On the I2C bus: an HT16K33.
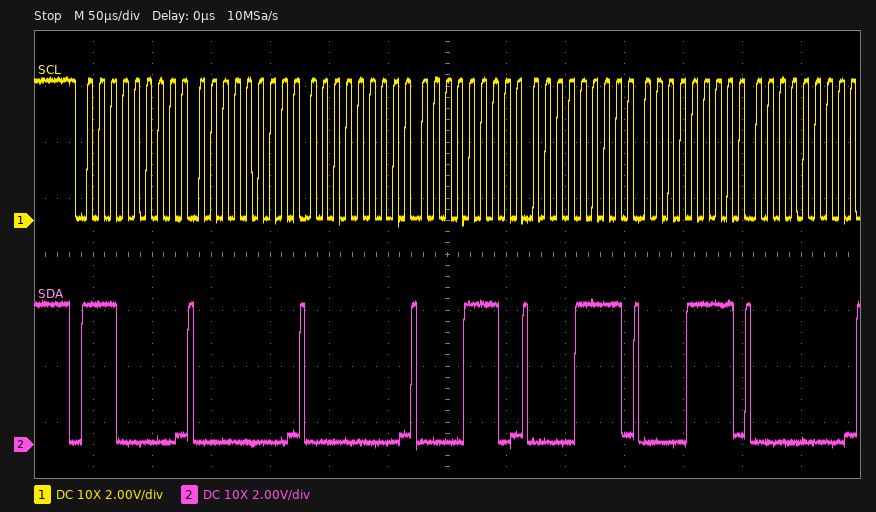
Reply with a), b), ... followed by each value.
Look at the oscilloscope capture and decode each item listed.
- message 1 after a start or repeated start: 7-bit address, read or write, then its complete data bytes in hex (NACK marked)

a) 0x70 write: 00 00 0E 0F 0F 00
